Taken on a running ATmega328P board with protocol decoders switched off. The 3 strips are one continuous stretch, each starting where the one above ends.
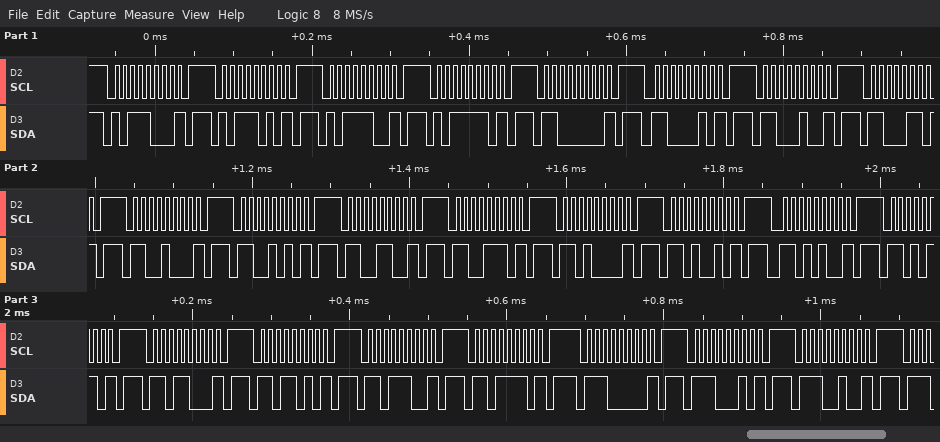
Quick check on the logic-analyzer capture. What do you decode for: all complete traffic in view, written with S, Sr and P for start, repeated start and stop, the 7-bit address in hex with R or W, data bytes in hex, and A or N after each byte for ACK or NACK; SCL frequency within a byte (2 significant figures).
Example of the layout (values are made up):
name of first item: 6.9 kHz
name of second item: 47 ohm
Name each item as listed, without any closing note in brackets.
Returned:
all complete traffic in view, written with S, Sr and P for start, repeated start and stop, the 7-bit address in hex with R or W, data bytes in hex, and A or N after each byte for ACK or NACK: S 5CW N P S 5DW N P S 5EW N P S 5FW N P S 60W N P S 61W N P S 62W N P S 63W N P S 64W N P S 65W N P S 66W N P S 67W N P S 68W N P S 69W N P S 6AW N P S 6BW N P S 6CW N P S 6DW N P S 6EW N P S 6FW N P S 70W N P S 71W N P S 72W N P
SCL frequency within a byte: 100 kHz
